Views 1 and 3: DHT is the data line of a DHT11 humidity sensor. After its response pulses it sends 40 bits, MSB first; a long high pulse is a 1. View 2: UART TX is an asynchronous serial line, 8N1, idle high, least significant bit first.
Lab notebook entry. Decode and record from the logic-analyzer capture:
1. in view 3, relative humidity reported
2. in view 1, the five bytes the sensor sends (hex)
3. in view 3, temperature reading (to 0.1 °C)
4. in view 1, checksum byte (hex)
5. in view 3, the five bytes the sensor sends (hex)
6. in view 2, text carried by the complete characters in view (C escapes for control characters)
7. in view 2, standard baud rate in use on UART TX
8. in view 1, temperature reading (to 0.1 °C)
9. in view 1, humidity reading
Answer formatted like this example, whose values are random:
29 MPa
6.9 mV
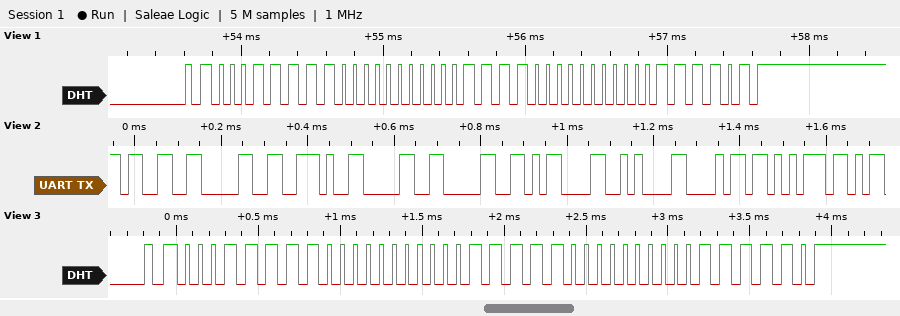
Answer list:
31 %
1F 00 1E 00 3D
31.0 °C
0x3D
1F 00 1F 00 3E
"30.00\r\nhu"
57600 baud
30.0 °C
31 %
